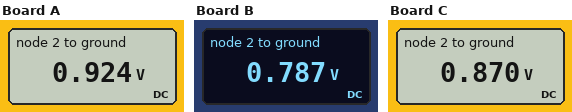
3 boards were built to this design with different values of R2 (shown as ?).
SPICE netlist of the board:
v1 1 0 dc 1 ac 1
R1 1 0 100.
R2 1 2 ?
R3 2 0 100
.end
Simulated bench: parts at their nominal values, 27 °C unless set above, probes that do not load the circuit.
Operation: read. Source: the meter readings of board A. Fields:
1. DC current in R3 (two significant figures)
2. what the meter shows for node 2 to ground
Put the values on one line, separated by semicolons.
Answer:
9.2 mA; 0.924 V
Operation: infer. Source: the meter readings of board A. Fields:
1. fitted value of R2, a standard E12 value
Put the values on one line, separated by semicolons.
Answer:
8.2 Ω
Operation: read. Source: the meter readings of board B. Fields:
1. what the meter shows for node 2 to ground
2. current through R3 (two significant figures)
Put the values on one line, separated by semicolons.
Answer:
0.787 V; 7.9 mA
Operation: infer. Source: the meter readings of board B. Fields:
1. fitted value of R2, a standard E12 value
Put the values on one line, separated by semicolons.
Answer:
27 Ω
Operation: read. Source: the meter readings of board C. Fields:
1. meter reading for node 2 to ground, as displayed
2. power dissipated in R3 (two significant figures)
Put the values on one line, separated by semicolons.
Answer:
0.870 V; 7.6 mW
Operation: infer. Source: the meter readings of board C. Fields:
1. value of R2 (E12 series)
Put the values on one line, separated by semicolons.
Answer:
15 Ω
